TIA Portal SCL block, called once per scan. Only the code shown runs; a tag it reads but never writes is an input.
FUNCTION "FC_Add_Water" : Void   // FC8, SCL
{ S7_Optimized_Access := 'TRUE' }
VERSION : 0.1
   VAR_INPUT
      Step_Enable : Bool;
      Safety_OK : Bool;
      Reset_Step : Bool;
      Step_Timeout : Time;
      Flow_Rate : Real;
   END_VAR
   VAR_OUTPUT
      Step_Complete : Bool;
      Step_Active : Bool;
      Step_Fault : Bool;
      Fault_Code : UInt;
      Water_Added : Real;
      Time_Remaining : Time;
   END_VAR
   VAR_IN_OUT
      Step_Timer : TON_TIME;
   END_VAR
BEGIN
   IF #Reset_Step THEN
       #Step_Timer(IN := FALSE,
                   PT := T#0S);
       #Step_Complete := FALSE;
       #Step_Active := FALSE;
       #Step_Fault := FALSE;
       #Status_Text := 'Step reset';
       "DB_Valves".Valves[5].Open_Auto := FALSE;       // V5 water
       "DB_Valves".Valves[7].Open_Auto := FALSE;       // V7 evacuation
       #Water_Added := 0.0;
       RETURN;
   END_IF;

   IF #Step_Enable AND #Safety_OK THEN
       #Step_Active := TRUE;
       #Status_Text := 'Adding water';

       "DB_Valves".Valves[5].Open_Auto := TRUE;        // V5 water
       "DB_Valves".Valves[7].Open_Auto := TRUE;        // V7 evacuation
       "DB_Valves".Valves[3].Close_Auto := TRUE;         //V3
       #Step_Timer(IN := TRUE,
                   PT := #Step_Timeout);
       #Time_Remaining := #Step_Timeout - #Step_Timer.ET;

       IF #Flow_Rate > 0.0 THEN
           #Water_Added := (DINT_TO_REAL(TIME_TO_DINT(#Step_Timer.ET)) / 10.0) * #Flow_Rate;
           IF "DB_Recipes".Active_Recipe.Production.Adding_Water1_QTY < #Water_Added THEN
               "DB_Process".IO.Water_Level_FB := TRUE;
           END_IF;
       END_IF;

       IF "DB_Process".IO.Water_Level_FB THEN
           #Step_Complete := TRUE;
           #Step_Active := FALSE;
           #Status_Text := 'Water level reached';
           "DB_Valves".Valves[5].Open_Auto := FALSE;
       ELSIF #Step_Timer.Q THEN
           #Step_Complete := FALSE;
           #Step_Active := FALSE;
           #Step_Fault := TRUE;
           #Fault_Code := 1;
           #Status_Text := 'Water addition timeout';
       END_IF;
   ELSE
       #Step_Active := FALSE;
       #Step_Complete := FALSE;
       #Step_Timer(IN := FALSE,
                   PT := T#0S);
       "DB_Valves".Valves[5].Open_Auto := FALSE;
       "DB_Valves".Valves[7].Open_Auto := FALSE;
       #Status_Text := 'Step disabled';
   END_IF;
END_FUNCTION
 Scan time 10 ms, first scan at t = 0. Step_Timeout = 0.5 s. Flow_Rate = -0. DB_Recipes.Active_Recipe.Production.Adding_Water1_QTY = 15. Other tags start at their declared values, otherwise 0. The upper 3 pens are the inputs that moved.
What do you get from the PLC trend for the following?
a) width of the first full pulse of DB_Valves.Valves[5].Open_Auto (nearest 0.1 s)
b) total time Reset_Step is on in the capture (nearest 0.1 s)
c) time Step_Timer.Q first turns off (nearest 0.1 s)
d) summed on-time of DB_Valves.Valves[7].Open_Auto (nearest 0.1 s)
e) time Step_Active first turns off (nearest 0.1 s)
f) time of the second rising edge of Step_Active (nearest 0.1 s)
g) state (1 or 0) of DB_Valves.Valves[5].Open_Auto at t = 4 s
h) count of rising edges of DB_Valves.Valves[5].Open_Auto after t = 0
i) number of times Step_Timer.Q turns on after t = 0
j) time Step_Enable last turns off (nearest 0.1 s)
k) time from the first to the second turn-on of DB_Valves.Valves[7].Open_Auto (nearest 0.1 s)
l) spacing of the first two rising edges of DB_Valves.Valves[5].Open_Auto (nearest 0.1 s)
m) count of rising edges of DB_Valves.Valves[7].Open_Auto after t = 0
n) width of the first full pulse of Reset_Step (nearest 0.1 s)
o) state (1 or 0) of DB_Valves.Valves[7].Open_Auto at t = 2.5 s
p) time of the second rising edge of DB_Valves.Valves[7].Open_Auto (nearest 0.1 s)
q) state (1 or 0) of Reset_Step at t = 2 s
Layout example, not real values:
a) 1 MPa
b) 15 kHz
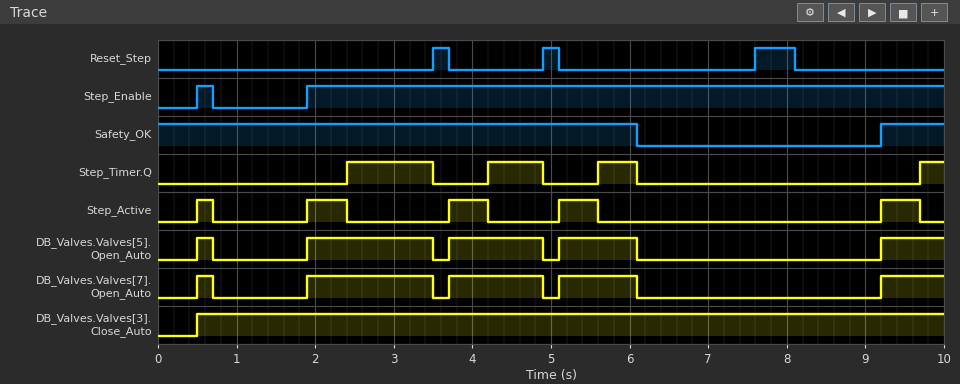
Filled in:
a) 0.2 s
b) 0.9 s
c) 3.5 s
d) 4.8 s
e) 0.7 s
f) 1.9 s
g) 1
h) 5
i) 4
j) 0.7 s
k) 1.4 s
l) 1.4 s
m) 5
n) 0.2 s
o) 1
p) 1.9 s
q) 0
